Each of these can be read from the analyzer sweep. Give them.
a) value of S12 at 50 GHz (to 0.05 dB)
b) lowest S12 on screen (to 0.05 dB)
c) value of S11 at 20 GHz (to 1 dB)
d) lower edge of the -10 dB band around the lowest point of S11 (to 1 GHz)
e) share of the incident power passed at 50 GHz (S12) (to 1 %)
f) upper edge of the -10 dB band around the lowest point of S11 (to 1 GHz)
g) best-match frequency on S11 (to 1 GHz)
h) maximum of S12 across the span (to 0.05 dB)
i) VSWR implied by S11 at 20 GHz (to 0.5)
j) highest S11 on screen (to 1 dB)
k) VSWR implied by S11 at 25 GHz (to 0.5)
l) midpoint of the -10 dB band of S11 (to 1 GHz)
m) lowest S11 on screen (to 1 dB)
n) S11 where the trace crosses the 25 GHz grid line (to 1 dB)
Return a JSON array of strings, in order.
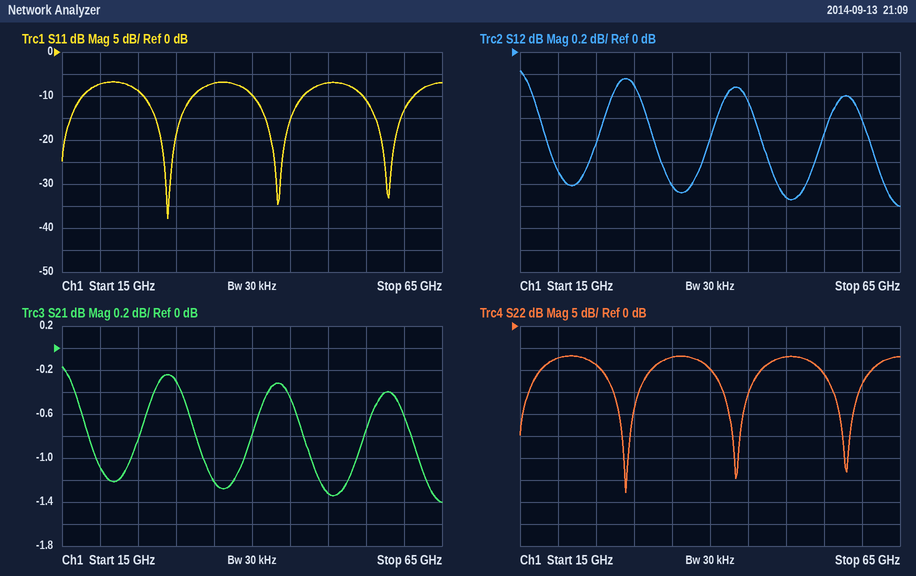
["-1.30 dB", "-1.40 dB", "-7 dB", "26 GHz", "74 %", "32 GHz", "29 GHz", "-0.15 dB", "2.5", "-7 dB", "2.0", "29 GHz", "-38 dB", "-9 dB"]
